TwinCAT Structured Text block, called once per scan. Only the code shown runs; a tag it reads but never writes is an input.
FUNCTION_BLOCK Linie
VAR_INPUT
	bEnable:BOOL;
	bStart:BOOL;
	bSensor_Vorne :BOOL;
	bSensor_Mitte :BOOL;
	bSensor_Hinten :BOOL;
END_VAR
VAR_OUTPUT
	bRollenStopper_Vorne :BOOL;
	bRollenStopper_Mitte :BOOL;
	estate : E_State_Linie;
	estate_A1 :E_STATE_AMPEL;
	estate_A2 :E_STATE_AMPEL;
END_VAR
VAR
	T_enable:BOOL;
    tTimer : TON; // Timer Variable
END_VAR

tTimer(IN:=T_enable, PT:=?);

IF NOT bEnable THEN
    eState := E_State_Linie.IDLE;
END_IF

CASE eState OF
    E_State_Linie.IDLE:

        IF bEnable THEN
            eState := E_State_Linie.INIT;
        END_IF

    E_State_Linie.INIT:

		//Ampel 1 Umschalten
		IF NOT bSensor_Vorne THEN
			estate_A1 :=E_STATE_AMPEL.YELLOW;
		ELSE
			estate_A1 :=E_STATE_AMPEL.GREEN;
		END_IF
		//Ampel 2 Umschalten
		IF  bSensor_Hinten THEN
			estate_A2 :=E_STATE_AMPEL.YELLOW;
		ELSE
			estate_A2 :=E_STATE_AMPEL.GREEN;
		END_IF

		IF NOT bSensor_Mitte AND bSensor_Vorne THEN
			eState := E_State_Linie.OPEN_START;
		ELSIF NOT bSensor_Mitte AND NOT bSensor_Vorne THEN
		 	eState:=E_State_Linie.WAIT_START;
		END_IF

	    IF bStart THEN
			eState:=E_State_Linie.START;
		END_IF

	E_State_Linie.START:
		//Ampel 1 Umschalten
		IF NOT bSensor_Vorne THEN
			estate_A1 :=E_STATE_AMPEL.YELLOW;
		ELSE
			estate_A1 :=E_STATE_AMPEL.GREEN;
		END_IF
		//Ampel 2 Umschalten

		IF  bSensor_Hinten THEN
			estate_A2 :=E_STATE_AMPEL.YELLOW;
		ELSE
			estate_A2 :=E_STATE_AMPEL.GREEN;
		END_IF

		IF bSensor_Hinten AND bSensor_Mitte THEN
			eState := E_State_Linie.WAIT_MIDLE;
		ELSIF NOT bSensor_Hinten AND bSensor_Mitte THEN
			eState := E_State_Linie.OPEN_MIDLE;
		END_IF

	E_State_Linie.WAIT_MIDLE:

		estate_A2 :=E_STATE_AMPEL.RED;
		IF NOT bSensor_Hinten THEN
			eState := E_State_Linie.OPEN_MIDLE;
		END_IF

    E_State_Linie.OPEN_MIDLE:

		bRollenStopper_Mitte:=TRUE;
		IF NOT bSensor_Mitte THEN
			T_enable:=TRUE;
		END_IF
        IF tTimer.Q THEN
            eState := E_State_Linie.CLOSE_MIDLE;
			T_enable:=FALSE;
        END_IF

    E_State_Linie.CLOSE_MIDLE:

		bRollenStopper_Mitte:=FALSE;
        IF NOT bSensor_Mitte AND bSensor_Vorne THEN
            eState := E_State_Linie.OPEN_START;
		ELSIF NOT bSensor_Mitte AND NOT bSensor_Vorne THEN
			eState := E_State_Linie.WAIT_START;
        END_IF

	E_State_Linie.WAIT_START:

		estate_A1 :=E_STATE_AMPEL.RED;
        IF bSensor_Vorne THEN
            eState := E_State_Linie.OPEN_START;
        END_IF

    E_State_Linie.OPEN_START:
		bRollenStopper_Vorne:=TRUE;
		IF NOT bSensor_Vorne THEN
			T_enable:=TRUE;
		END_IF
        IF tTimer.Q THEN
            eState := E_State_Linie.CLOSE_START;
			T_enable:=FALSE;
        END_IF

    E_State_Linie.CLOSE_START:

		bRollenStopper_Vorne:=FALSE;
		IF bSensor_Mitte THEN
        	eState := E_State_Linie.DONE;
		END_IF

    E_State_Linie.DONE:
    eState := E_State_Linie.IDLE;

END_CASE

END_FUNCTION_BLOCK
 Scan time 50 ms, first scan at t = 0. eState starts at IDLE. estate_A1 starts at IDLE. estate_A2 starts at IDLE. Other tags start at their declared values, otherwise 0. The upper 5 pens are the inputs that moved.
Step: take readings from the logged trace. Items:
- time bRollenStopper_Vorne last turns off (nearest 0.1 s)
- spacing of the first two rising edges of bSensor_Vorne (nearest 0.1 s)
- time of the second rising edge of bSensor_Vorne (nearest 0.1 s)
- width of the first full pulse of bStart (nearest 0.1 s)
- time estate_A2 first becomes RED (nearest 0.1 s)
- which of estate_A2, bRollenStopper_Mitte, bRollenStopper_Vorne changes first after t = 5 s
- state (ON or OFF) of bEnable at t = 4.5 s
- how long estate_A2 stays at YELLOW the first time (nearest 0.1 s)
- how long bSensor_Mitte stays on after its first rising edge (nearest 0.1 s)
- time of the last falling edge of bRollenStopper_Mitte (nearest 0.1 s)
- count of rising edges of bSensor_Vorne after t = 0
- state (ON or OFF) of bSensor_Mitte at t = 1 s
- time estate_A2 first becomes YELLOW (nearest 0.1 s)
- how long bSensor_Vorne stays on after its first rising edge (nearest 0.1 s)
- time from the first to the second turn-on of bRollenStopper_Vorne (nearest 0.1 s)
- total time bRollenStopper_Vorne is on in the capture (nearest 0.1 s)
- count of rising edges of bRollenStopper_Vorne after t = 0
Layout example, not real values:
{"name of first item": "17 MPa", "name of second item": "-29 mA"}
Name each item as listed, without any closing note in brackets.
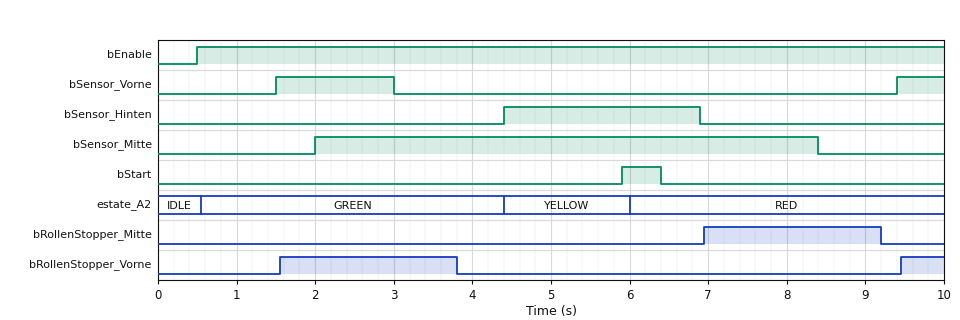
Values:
{"time bRollenStopper_Vorne last turns off": "3.8 s", "spacing of the first two rising edges of bSensor_Vorne": "7.9 s", "time of the second rising edge of bSensor_Vorne": "9.4 s", "width of the first full pulse of bStart": "0.5 s", "time estate_A2 first becomes RED": "6.0 s", "which of estate_A2, bRollenStopper_Mitte, bRollenStopper_Vorne changes first after t = 5 s": "estate_A2", "state (ON or OFF) of bEnable at t = 4.5 s": "ON", "how long estate_A2 stays at YELLOW the first time": "1.6 s", "how long bSensor_Mitte stays on after its first rising edge": "6.4 s", "time of the last falling edge of bRollenStopper_Mitte": "9.2 s", "count of rising edges of bSensor_Vorne after t = 0": "2", "state (ON or OFF) of bSensor_Mitte at t = 1 s": "OFF", "time estate_A2 first becomes YELLOW": "4.4 s", "how long bSensor_Vorne stays on after its first rising edge": "1.5 s", "time from the first to the second turn-on of bRollenStopper_Vorne": "7.9 s", "total time bRollenStopper_Vorne is on in the capture": "2.8 s", "count of rising edges of bRollenStopper_Vorne after t = 0": "2"}
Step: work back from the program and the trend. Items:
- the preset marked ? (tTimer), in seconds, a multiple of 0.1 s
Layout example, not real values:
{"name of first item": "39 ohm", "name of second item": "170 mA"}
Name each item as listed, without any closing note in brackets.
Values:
{"the preset marked ? (tTimer), in seconds, a multiple of 0.1 s": "0.7 s"}
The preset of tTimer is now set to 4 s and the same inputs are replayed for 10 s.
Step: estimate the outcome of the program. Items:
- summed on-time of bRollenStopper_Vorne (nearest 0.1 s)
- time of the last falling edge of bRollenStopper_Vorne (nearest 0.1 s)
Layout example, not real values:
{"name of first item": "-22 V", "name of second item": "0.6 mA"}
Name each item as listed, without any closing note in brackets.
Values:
{"summed on-time of bRollenStopper_Vorne": "6.1 s", "time of the last falling edge of bRollenStopper_Vorne": "7.1 s"}
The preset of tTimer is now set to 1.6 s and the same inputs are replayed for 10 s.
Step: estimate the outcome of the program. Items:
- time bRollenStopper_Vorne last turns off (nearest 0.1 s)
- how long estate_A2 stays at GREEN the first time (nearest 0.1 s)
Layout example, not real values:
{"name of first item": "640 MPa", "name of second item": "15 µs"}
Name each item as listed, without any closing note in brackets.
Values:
{"time bRollenStopper_Vorne last turns off": "4.7 s", "how long estate_A2 stays at GREEN the first time": "4.3 s"}
